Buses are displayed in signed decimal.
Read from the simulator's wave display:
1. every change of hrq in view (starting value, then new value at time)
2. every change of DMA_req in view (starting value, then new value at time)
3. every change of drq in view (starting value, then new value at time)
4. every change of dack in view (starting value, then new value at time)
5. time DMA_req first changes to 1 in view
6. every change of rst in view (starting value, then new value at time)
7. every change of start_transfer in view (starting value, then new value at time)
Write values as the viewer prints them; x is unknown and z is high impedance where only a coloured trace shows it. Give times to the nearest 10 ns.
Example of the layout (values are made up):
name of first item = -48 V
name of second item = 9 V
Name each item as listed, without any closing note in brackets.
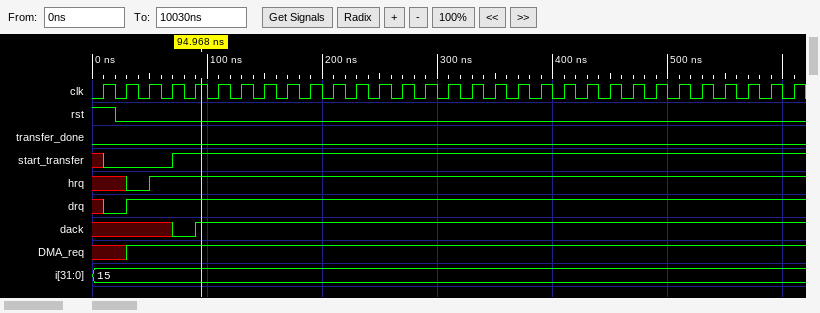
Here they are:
every change of hrq in view = x, 0 at 30 ns, 1 at 50 ns
every change of DMA_req in view = x, 1 at 30 ns
every change of drq in view = x, 0 at 10 ns, 1 at 30 ns
every change of dack in view = x, 0 at 70 ns, 1 at 90 ns
time DMA_req first changes to 1 in view = 30 ns
every change of rst in view = 1, 0 at 20 ns
every change of start_transfer in view = x, 0 at 10 ns, 1 at 70 ns
